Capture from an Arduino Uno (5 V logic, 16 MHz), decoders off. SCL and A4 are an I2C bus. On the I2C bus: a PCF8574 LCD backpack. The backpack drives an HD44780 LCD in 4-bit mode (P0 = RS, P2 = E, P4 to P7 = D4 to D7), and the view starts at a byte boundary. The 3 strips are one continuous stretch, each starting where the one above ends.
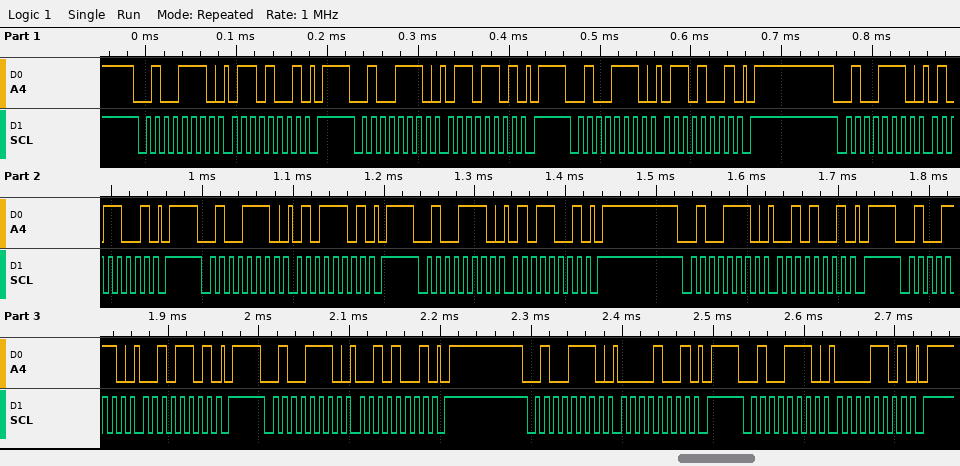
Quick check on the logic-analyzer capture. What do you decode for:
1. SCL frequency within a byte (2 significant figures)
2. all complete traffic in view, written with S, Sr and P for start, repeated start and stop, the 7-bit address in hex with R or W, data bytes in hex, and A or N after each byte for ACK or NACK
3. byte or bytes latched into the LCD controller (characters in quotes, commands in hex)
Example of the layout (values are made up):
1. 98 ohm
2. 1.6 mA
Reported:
1. 100 kHz
2. S 27W A 69 A P S 27W A 6D A P S 27W A 69 A P S 27W A 59 A P S 27W A 5D A P S 27W A 59 A P S 27W A 29 A P S 27W A 2D A P S 27W A 29 A P S 27W A 09 A P S 27W A 0D A P
3. 'e'
